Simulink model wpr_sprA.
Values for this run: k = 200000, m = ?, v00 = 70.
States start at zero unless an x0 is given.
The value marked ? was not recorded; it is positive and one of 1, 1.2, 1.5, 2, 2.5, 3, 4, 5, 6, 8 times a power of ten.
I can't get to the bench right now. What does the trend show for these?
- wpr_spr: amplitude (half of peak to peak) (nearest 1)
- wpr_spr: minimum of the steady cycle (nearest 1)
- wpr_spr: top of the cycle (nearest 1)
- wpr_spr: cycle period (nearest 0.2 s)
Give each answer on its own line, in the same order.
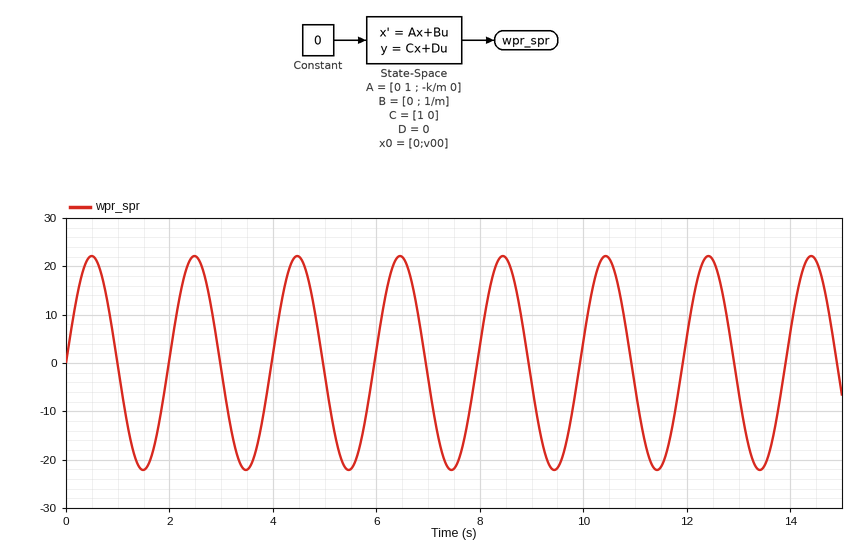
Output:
22
-22
22
2.0 s
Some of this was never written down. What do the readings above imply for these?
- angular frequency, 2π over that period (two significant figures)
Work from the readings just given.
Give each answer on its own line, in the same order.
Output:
3.1 rad/s
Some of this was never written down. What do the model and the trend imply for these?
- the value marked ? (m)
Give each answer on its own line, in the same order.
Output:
20000
